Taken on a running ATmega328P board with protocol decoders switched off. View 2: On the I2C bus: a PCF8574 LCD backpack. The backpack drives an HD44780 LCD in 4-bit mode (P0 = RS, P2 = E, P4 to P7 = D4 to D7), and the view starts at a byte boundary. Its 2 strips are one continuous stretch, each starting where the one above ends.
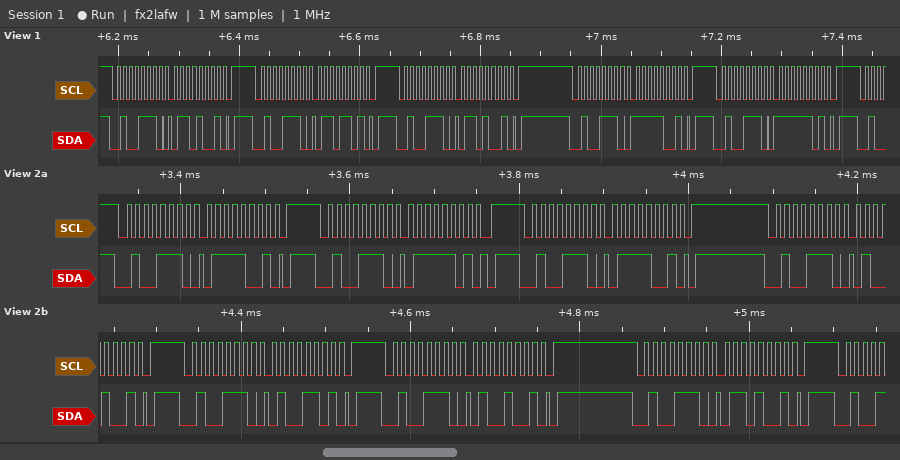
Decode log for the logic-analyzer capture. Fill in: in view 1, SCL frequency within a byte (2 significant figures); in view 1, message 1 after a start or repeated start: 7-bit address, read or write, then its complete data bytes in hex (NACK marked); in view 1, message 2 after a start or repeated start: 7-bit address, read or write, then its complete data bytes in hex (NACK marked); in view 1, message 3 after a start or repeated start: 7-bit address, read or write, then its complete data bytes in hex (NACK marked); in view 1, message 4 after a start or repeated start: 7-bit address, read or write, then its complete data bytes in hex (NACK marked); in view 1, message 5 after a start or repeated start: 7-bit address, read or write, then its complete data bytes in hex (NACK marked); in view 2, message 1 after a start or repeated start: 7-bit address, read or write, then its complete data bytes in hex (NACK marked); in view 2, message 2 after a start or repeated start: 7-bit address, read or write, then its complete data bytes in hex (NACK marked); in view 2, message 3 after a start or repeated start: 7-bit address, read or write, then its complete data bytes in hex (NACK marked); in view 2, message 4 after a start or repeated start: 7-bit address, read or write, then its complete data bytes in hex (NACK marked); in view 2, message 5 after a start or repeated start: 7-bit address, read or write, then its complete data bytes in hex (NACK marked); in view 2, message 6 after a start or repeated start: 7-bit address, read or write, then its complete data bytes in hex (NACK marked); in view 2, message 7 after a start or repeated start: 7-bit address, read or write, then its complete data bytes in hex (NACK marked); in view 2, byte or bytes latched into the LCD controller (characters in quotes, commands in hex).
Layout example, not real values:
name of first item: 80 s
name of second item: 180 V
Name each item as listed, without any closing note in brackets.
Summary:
in view 1, SCL frequency within a byte: 100 kHz
in view 1, message 1 after a start or repeated start: 7-bit address, read or write, then its complete data bytes in hex: 0x27 write: 69
in view 1, message 2 after a start or repeated start: 7-bit address, read or write, then its complete data bytes in hex: 0x27 write: 6D
in view 1, message 3 after a start or repeated start: 7-bit address, read or write, then its complete data bytes in hex: 0x27 write: 69
in view 1, message 4 after a start or repeated start: 7-bit address, read or write, then its complete data bytes in hex: 0x27 write: F9
in view 1, message 5 after a start or repeated start: 7-bit address, read or write, then its complete data bytes in hex: 0x27 write: FD
in view 2, message 1 after a start or repeated start: 7-bit address, read or write, then its complete data bytes in hex: 0x27 write: 79
in view 2, message 2 after a start or repeated start: 7-bit address, read or write, then its complete data bytes in hex: 0x27 write: 7D
in view 2, message 3 after a start or repeated start: 7-bit address, read or write, then its complete data bytes in hex: 0x27 write: 79
in view 2, message 4 after a start or repeated start: 7-bit address, read or write, then its complete data bytes in hex: 0x27 write: 49
in view 2, message 5 after a start or repeated start: 7-bit address, read or write, then its complete data bytes in hex: 0x27 write: 4D
in view 2, message 6 after a start or repeated start: 7-bit address, read or write, then its complete data bytes in hex: 0x27 write: 49
in view 2, message 7 after a start or repeated start: 7-bit address, read or write, then its complete data bytes in hex: 0x27 write: 69
in view 2, byte or bytes latched into the LCD controller: 't'
